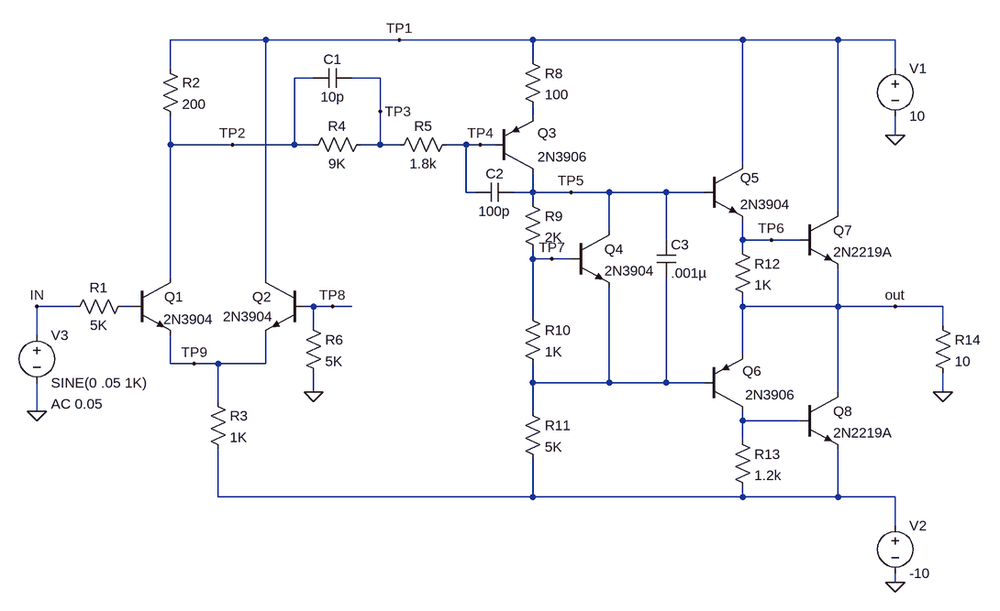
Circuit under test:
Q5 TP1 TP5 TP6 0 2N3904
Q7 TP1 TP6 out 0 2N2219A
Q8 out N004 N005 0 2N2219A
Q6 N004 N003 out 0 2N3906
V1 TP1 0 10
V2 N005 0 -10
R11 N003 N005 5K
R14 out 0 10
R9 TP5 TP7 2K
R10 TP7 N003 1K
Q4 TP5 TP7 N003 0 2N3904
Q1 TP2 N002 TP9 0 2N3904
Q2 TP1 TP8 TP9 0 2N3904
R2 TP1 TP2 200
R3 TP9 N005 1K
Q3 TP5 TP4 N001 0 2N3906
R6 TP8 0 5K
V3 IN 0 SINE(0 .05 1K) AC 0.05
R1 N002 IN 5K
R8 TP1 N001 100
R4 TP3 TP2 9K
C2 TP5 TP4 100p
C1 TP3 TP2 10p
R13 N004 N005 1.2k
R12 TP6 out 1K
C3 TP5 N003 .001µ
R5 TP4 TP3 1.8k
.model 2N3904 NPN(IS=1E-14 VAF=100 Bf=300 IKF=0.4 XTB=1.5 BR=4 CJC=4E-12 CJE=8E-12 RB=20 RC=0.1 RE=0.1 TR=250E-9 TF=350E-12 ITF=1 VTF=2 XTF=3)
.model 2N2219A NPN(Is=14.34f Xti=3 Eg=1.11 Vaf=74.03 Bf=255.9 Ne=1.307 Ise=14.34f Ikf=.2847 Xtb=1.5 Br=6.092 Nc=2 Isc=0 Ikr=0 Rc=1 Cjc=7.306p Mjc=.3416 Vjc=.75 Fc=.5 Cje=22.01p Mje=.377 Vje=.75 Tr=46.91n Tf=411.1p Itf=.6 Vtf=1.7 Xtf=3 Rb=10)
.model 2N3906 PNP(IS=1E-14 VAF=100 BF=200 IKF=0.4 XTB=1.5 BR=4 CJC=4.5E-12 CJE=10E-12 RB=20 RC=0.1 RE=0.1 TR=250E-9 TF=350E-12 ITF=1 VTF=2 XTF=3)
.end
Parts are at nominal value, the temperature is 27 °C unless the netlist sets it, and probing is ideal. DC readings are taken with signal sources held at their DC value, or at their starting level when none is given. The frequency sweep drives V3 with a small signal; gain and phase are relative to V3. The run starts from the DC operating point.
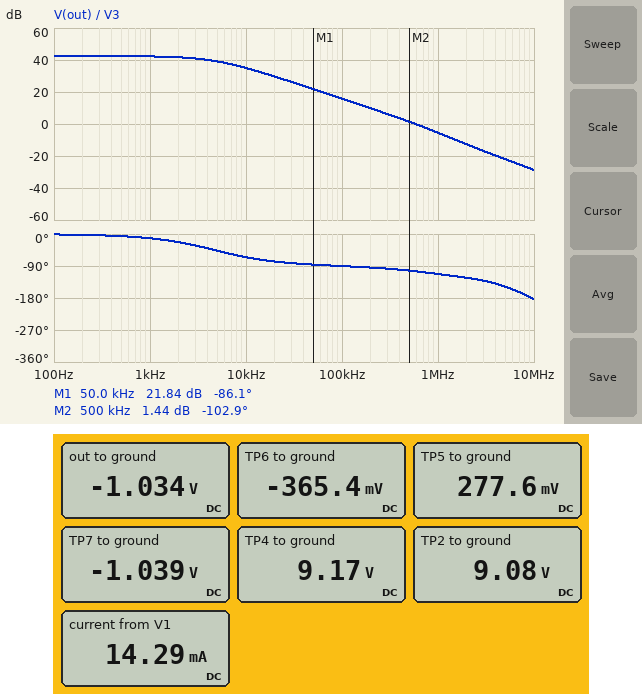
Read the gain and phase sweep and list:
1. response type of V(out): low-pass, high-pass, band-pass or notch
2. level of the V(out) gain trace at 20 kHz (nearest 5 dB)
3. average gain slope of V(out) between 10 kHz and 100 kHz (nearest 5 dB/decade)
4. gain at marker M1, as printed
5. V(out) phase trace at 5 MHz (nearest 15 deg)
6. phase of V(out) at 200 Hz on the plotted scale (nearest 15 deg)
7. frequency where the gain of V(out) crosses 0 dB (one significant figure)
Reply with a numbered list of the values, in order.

1. low-pass
2. 30 dB
3. -20 dB/decade
4. 21.84 dB
5. -150 deg
6. 0 deg
7. 600 kHz
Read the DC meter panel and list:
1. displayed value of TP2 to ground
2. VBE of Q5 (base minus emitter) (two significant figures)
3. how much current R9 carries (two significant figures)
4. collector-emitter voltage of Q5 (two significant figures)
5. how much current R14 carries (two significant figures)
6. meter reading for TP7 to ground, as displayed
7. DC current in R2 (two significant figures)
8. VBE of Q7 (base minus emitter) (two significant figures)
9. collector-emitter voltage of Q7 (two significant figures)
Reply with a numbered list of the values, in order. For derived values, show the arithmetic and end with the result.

1. 9.08 V
2. 277.6 mV - (-365.4 mV) = 640 mV
3. (277.6 mV - (-1.039 V)) / 2 kΩ = 660 µA
4. 10 V - (-365.4 mV) = 10 V
5. (0 V - (-1.034 V)) / 10 Ω = 100 mA
6. -1.039 V
7. (10 V - 9.08 V) / 200 Ω = 4.6 mA
8. -365.4 mV - (-1.034 V) = 670 mV
9. 10 V - (-1.034 V) = 11 V
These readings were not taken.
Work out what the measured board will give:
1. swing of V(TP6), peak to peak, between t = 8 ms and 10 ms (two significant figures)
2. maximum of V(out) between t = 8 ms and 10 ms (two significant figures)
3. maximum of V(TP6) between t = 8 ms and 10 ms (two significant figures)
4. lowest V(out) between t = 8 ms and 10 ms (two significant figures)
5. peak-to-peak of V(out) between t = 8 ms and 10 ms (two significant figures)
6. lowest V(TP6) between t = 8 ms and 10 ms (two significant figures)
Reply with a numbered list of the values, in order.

1. 13 V
2. 5.3 V
3. 6.2 V
4. -6.9 V
5. 12 V
6. -6.9 V
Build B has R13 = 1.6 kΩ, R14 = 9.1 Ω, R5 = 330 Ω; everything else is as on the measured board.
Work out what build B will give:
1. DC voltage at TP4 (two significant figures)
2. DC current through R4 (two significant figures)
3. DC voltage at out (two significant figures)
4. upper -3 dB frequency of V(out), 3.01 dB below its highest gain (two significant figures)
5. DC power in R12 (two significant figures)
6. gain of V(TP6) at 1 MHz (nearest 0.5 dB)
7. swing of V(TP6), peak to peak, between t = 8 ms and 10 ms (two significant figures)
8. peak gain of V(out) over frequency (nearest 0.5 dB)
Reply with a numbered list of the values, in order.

1. 9.2 V
2. 8.0 µA
3. -710 mV
4. 5.2 kHz
5. 460 µW
6. -4.0 dB
7. 14 V
8. 43.0 dB
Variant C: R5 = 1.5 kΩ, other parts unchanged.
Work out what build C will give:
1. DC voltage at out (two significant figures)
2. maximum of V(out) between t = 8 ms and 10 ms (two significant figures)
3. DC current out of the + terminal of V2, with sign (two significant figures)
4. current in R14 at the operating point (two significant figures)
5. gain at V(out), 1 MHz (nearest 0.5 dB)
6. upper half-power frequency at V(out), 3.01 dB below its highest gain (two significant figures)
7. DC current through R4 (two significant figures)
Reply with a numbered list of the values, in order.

1. -970 mV
2. 5.4 V
3. -110 mA
4. 97 mA
5. -5.0 dB
6. 4.8 kHz
7. 7.7 µA
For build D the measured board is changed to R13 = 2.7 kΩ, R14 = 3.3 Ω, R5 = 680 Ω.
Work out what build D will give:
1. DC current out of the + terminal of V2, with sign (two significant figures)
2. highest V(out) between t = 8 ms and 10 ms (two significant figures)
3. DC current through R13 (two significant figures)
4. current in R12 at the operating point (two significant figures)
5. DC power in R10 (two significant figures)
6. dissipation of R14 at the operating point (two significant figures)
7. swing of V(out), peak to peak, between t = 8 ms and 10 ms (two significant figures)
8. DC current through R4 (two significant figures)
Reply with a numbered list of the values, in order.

1. -240 mA
2. 4.9 V
3. 300 µA
4. 660 µA
5. 430 µW
6. 170 mW
7. 11 V
8. 7.9 µA
